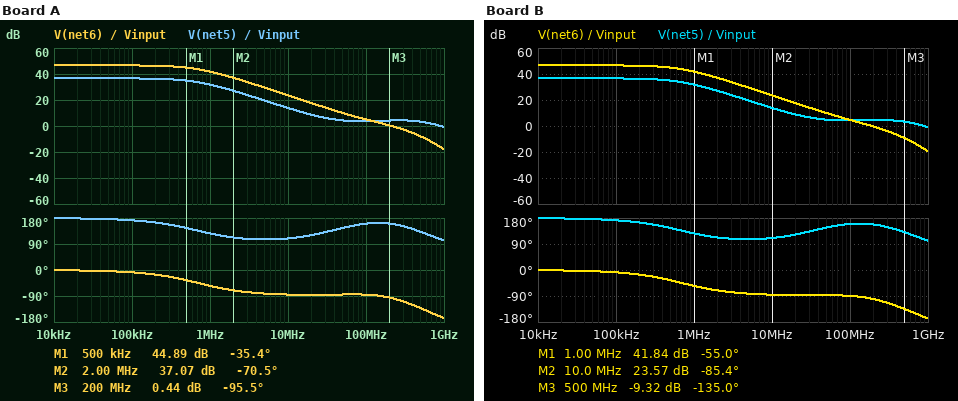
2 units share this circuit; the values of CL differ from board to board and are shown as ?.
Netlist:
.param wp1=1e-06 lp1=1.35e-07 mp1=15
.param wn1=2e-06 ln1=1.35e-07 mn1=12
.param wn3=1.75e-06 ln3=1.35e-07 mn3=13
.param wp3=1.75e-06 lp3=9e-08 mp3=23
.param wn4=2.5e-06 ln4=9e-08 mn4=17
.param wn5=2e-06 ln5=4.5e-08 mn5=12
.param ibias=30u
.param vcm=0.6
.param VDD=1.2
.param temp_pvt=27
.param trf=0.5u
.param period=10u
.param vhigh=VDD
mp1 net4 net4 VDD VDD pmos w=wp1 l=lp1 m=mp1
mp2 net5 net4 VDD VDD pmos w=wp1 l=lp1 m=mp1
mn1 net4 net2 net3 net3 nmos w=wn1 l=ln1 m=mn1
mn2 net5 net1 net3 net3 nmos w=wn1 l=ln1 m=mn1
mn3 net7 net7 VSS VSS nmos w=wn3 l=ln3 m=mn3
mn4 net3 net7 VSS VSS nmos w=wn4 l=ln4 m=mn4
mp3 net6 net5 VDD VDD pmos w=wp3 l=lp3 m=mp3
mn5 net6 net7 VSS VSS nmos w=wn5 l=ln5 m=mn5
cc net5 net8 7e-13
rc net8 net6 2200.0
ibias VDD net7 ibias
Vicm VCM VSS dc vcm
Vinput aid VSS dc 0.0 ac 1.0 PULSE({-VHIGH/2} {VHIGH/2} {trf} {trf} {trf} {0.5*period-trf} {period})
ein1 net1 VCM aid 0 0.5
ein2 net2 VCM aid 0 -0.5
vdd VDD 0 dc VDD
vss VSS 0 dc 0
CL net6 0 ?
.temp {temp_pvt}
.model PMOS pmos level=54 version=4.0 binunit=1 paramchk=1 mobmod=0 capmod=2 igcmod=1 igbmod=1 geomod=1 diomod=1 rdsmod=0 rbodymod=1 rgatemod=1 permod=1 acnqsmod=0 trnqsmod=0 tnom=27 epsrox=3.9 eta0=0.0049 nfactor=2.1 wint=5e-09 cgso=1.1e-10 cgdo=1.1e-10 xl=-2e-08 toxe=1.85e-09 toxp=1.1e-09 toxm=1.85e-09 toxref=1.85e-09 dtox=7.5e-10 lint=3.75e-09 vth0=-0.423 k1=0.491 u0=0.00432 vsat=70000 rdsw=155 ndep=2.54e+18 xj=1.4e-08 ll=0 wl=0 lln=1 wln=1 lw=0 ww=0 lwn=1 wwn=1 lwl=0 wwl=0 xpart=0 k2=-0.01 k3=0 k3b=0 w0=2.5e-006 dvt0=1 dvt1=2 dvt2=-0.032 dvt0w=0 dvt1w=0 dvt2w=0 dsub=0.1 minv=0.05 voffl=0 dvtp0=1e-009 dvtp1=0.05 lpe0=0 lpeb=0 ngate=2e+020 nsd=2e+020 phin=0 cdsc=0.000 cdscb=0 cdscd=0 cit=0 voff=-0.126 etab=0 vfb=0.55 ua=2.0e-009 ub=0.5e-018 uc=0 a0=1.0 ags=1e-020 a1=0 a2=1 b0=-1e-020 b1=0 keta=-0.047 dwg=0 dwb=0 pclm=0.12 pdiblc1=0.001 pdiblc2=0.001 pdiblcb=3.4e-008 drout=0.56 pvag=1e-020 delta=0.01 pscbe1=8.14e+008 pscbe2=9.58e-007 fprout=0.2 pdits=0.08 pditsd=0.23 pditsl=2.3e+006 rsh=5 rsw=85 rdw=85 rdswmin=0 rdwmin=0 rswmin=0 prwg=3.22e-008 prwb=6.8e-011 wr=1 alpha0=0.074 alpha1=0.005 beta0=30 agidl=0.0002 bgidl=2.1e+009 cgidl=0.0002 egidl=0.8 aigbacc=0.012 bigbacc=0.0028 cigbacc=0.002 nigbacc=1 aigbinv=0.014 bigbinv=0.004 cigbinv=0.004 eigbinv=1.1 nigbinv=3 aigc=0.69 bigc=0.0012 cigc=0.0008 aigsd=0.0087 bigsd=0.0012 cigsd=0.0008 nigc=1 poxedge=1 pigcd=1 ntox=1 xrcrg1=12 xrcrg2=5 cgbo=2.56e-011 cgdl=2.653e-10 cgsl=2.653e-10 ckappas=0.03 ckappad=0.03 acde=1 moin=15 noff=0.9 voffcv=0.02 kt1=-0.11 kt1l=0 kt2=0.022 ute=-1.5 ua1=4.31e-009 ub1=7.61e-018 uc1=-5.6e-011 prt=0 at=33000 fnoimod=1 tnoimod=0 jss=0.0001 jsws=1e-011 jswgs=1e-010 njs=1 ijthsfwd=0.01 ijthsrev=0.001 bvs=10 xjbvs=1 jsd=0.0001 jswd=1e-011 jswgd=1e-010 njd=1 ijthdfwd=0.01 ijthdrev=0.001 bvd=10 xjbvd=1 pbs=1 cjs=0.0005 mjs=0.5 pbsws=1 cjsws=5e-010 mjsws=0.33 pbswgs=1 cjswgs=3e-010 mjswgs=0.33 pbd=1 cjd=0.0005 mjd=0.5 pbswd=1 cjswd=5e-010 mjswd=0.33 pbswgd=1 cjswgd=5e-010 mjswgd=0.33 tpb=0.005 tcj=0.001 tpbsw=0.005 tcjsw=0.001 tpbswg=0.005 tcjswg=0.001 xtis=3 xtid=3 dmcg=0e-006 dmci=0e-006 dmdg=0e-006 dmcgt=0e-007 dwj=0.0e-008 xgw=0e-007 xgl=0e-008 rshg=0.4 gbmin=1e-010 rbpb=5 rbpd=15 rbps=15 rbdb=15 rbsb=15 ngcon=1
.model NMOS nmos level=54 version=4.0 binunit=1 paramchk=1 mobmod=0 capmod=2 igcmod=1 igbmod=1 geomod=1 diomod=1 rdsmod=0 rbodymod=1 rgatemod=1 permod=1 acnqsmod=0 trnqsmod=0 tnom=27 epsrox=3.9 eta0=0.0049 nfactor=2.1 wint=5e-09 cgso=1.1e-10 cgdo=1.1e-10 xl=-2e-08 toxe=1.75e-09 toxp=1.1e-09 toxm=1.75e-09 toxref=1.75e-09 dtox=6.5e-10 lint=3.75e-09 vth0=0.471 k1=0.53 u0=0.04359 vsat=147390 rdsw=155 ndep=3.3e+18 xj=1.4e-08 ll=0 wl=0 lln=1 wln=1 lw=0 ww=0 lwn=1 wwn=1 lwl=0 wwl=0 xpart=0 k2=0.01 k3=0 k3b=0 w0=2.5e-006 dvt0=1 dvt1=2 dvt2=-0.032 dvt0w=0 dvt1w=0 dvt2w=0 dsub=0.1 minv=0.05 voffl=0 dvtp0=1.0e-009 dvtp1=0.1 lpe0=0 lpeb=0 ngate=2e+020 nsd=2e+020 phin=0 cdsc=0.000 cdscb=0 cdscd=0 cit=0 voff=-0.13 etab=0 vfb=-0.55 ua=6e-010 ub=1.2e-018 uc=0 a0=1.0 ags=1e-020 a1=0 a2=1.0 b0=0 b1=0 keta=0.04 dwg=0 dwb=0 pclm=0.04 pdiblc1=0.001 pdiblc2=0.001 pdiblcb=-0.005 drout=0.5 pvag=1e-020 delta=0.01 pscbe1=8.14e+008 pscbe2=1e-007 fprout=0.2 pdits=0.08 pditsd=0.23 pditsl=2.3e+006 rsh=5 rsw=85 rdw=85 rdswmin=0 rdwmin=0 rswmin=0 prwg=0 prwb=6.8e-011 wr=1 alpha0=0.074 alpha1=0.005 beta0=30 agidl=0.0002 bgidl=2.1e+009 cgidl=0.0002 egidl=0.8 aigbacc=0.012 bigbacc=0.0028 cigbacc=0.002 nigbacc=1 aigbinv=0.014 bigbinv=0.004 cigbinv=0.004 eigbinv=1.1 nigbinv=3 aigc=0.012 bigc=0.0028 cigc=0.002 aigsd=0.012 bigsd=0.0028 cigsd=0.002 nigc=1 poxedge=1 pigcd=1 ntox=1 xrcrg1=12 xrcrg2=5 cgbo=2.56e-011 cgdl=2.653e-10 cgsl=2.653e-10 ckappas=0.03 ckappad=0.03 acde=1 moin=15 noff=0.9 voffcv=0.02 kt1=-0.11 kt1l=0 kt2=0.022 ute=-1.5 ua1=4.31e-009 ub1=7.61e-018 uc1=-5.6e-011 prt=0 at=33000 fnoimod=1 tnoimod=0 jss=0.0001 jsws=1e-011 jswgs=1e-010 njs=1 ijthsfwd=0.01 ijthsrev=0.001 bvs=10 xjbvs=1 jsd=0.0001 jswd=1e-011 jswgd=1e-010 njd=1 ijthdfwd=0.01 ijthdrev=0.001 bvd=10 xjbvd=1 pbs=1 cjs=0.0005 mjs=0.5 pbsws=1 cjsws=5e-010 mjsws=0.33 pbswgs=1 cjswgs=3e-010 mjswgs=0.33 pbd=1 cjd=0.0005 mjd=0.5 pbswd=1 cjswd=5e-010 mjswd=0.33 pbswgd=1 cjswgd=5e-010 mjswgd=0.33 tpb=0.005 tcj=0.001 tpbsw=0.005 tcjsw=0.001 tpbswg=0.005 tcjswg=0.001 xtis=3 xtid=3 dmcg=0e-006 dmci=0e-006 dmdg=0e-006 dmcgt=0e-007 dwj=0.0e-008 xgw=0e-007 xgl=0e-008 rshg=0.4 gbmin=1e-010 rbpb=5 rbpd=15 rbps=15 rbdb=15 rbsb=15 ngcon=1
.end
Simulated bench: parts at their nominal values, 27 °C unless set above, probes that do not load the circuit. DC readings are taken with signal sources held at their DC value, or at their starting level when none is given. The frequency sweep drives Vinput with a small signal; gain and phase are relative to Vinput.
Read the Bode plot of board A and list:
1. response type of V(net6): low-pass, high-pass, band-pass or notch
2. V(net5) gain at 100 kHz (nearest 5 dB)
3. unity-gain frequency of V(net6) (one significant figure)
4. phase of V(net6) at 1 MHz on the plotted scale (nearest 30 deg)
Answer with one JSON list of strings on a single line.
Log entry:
["low-pass", "35 dB", "200 MHz", "-60 deg"]
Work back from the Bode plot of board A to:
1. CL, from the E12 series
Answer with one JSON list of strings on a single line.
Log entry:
["3.3 pF"]
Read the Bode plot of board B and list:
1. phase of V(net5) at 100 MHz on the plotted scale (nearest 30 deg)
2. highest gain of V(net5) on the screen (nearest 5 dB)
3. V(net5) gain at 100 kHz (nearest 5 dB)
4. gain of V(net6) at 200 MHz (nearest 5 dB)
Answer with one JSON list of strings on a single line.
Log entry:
["150 deg", "35 dB", "35 dB", "0 dB"]
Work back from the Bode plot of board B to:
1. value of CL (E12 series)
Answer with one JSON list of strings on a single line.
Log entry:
["3.9 pF"]
